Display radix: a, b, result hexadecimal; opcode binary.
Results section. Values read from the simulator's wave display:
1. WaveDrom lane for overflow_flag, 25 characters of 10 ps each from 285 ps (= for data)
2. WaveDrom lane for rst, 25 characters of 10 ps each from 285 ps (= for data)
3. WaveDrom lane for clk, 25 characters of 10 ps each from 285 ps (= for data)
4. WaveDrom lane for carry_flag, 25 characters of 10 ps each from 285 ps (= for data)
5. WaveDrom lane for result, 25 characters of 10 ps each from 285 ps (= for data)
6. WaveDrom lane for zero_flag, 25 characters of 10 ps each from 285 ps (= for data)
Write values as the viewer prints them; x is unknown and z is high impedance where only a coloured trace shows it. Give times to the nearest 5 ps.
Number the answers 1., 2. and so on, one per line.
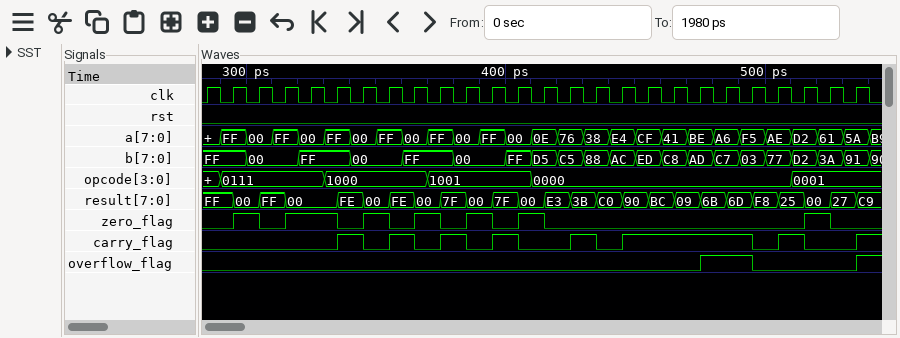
1. {name: 'overflow_flag', wave: '0..................1.0...'}
2. {name: 'rst', wave: '0........................'}
3. {name: 'clk', wave: 'p........................'}
4. {name: 'carry_flag', wave: '0....10101010.101....010.'}
5. {name: 'result', wave: '====.====================', data: 'FF 00 FF 00 FE 00 FE 00 7F 00 7F 00 E3 3B C0 90 BC 09 6B 6D F8 25 00 27'}
6. {name: 'zero_flag', wave: '0101.010101010.........10'}
